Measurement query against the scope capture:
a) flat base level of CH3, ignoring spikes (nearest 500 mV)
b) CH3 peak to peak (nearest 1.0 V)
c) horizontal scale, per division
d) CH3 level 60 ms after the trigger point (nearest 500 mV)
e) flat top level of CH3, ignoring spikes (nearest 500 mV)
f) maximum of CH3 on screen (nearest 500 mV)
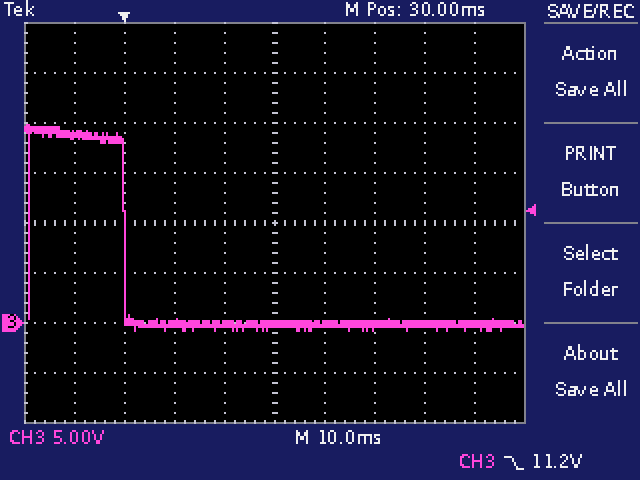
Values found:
0.0 V
21.0 V
10 ms
0.0 V
19.0 V
20.0 V
